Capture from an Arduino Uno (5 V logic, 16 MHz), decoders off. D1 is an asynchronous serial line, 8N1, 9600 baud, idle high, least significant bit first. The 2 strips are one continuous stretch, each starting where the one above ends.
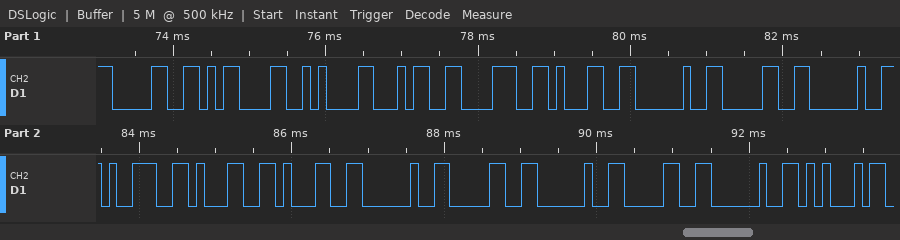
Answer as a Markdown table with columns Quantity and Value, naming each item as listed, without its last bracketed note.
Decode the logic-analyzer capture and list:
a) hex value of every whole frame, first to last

| Quantity | Value |
|---|---|
| hex value of every whole frame, first to last | 0x30 0x0D 0x0A 0x34 0x38 0x31 0x20 0x30 0x20 0x39 0x31 0x31 0x20 0x30 0x20 0x30 0x20 0x45 |
